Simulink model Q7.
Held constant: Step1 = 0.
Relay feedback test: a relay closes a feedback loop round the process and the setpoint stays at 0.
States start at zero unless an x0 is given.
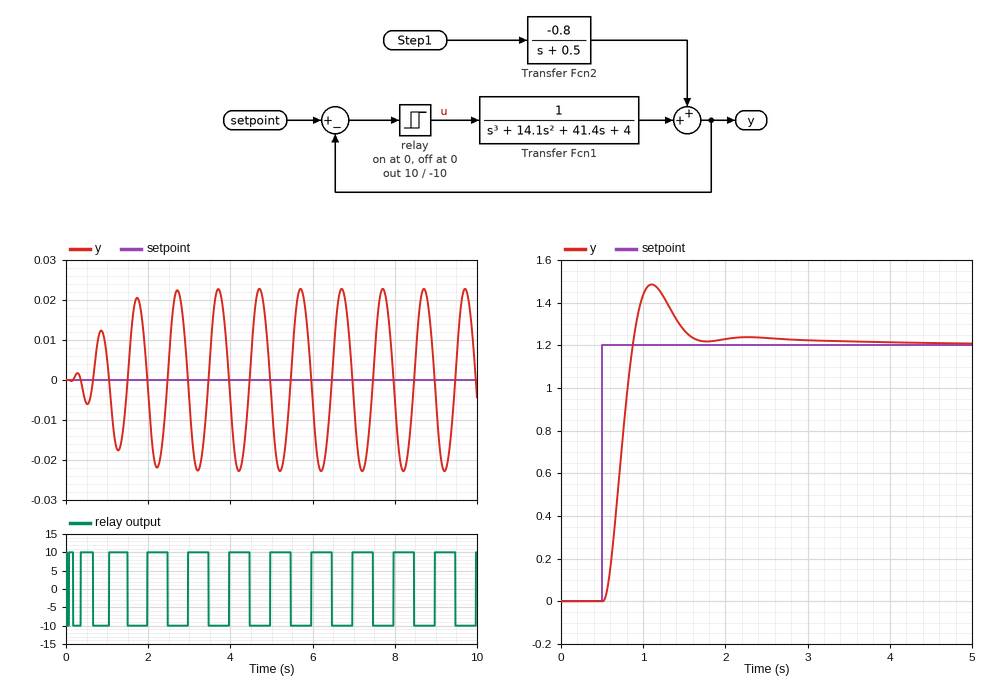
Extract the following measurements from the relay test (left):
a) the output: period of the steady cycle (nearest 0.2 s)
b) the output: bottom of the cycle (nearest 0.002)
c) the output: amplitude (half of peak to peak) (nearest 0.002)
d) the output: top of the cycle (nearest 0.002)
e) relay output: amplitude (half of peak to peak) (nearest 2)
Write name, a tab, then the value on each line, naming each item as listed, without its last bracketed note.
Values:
the output: period of the steady cycle	1.0 s
the output: bottom of the cycle	-0.022
the output: amplitude (half of peak to peak)	0.022
the output: top of the cycle	0.022
relay output: amplitude (half of peak to peak)	10
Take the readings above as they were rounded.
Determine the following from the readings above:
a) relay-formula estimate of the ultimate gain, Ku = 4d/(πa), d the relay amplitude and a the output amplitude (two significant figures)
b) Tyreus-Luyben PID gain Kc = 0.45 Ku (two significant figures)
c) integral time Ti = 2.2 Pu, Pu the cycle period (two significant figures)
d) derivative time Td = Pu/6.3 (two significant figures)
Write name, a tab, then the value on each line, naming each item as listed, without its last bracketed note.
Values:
relay-formula estimate of the ultimate gain, Ku = 4d/(πa), d the relay amplitude and a the output amplitude	580
Tyreus-Luyben PID gain Kc = 0.45 Ku	260
integral time Ti = 2.2 Pu, Pu the cycle period	2.2 s
derivative time Td = Pu/6.3	0.16 s
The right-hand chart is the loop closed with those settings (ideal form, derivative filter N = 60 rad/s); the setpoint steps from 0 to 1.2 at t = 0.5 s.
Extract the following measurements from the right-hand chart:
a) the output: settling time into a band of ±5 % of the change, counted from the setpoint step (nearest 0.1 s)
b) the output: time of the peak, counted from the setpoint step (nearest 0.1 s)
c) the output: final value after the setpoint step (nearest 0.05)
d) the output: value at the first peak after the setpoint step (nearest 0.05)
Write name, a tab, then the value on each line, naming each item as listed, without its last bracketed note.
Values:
the output: settling time into a band of ±5 % of the change, counted from the setpoint step	1.0 s
the output: time of the peak, counted from the setpoint step	0.6 s
the output: final value after the setpoint step	1.20
the output: value at the first peak after the setpoint step	1.50
